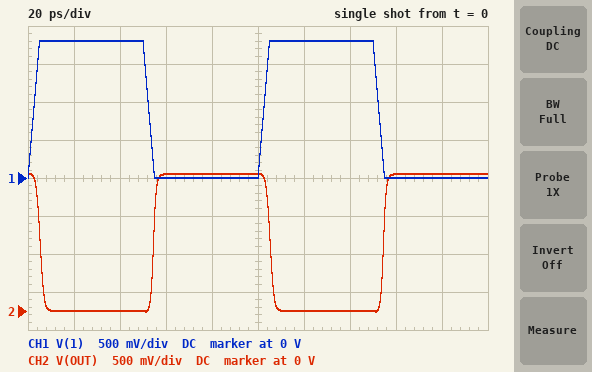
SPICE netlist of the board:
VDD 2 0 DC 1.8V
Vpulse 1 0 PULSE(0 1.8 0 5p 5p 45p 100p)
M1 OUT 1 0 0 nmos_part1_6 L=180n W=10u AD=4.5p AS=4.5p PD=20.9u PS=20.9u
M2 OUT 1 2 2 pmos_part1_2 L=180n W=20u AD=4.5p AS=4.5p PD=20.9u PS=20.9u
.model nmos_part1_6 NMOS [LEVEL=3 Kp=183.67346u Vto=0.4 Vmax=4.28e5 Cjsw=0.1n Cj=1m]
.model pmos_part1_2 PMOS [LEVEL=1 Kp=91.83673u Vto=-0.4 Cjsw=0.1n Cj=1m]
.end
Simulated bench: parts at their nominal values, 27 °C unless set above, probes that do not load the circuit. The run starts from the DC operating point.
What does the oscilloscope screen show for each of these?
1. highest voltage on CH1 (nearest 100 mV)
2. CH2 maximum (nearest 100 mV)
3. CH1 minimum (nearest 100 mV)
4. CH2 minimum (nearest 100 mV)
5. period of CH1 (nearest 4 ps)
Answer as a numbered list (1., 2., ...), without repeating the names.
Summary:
1. 1.8 V
2. 1.8 V
3. 0 V
4. 0 V
5. 100 ps
